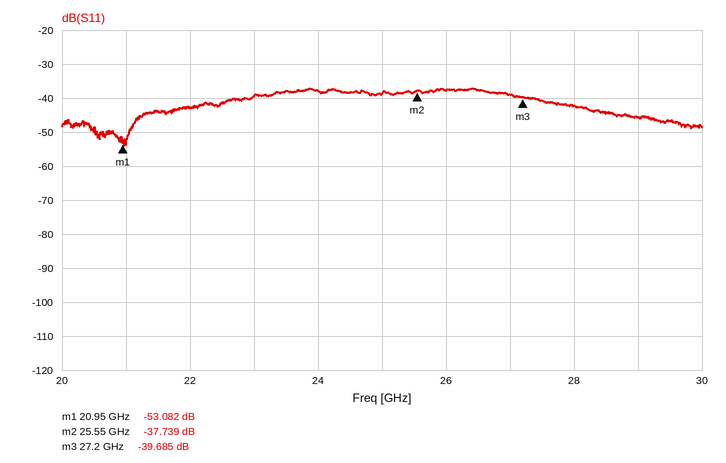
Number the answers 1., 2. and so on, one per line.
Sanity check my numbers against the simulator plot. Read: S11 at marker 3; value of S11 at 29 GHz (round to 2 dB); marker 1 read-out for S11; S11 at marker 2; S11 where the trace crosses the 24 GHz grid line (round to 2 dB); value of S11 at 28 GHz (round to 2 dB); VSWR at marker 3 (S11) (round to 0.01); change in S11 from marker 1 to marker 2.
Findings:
1. -39.685 dB
2. -46 dB
3. -53.082 dB
4. -37.739 dB
5. -38 dB
6. -42 dB
7. 1.02
8. 15.343 dB
